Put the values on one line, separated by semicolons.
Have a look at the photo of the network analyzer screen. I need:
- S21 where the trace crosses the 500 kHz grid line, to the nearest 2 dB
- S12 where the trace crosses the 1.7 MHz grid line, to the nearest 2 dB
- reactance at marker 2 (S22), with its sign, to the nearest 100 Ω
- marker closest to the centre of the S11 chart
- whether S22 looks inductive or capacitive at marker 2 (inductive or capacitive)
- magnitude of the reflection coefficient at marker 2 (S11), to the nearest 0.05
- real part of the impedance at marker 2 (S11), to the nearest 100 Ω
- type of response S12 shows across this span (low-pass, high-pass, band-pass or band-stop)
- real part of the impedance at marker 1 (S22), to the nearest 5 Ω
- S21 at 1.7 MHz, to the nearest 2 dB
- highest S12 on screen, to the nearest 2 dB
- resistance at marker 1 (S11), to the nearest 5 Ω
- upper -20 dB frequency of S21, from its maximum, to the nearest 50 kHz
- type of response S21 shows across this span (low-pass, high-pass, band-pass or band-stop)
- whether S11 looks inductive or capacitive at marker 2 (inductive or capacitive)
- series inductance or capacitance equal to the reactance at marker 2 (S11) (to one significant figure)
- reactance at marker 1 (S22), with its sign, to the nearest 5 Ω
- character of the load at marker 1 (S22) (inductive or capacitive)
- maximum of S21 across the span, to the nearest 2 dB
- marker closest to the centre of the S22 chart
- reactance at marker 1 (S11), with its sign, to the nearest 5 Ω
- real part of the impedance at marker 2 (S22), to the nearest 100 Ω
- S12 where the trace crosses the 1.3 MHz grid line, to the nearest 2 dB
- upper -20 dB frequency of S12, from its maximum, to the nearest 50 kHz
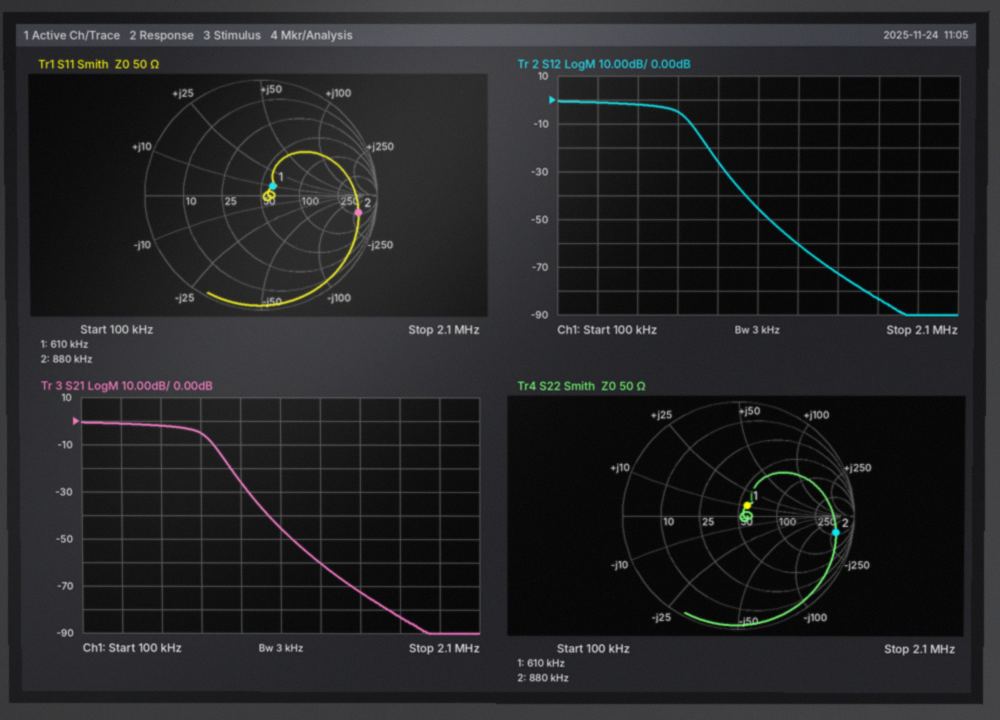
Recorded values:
-2 dB; -84 dB; -300 Ω; marker 1; capacitive; 0.85; 300 Ω; low-pass; 55 Ω; -84 dB; 0 dB; 60 Ω; 850 kHz; low-pass; capacitive; 600 pF; +10 Ω; inductive; 0 dB; marker 1; +10 Ω; 300 Ω; -60 dB; 850 kHz
